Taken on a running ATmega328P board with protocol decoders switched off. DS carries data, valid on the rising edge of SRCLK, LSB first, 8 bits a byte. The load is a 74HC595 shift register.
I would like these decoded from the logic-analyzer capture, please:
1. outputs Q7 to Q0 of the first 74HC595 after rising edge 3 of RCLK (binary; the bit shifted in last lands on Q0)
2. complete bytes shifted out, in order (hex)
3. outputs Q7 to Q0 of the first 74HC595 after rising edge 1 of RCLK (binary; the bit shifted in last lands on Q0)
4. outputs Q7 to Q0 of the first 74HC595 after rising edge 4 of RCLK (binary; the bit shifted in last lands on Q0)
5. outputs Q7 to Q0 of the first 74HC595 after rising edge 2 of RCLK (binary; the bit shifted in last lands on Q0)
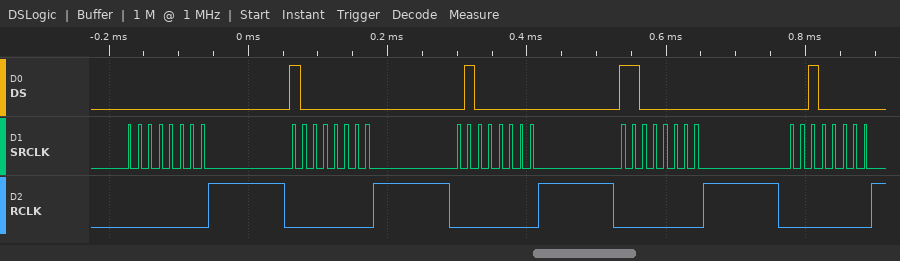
01000000
0x00 0x01 0x02 0x03 0x04
00000000
11000000
10000000
